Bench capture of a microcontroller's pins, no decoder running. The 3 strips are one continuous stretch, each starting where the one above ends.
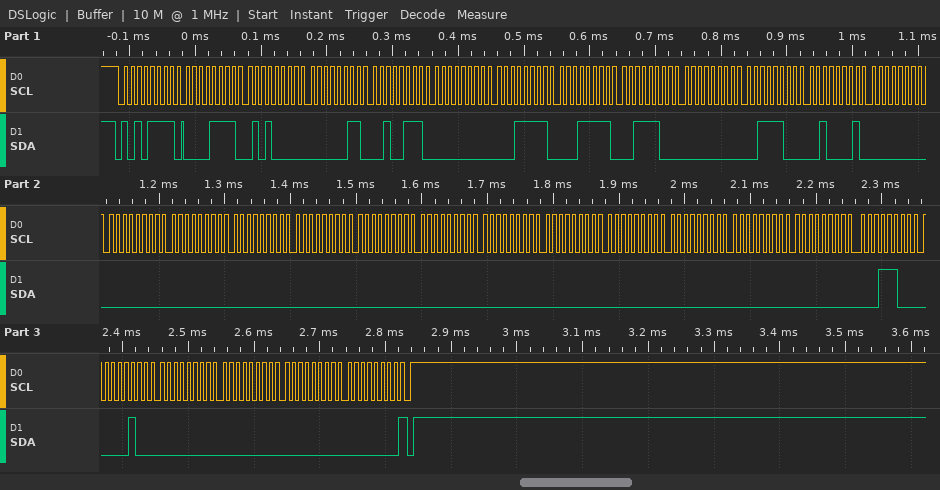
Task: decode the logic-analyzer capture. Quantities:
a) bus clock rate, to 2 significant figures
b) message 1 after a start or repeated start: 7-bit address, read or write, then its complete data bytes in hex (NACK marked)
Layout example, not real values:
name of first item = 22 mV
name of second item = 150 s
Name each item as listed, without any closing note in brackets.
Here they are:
bus clock rate, to 2 significant figures = 100 kHz
message 1 after a start or repeated start: 7-bit address, read or write, then its complete data bytes in hex = 0x57 read: 0F 50 03 27 00 1F 1F 3C 00 3C 21 00 00 00 00 00 00 00 00 00 00 00 00 00 1C 04 00 00 00 00 NACK
